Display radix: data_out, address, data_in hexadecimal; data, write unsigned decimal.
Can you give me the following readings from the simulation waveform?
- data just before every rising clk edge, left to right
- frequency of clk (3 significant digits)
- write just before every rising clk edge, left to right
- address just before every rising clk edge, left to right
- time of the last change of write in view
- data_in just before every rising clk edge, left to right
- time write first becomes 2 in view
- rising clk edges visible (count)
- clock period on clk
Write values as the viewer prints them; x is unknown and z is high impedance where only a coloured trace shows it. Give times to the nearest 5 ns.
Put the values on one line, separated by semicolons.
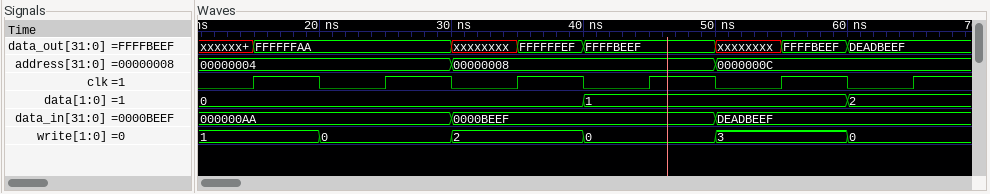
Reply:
0, 0, 0, 1, 1, 2; 100 MHz; 1, 0, 2, 0, 3, 0; 00000004, 00000004, 00000008, 00000008, 0000000C, 0000000C; 60 ns; 000000AA, 000000AA, 0000BEEF, 0000BEEF, DEADBEEF, DEADBEEF; 30 ns; 6; 10 ns
